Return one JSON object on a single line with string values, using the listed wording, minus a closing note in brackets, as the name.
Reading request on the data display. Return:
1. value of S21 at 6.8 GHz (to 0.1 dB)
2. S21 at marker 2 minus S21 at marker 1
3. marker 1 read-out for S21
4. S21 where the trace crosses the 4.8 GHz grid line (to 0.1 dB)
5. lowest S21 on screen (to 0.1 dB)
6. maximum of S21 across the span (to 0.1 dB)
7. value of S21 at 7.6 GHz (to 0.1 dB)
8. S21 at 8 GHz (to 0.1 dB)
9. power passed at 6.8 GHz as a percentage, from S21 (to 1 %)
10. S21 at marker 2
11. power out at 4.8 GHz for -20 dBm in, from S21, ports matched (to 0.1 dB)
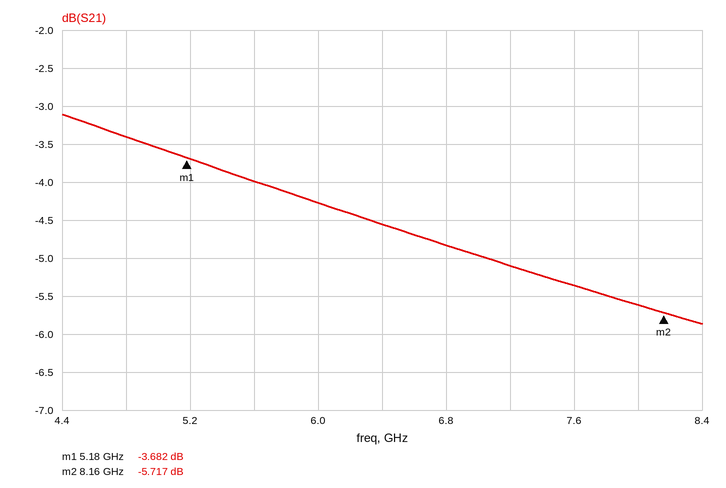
{"value of S21 at 6.8 GHz": "-4.8 dB", "S21 at marker 2 minus S21 at marker 1": "-2.035 dB", "marker 1 read-out for S21": "-3.682 dB", "S21 where the trace crosses the 4.8 GHz grid line": "-3.4 dB", "lowest S21 on screen": "-5.9 dB", "maximum of S21 across the span": "-3.1 dB", "value of S21 at 7.6 GHz": "-5.4 dB", "S21 at 8 GHz": "-5.6 dB", "power passed at 6.8 GHz as a percentage, from S21": "33 %", "S21 at marker 2": "-5.717 dB", "power out at 4.8 GHz for -20 dBm in, from S21, ports matched": "-23.4 dBm"}
